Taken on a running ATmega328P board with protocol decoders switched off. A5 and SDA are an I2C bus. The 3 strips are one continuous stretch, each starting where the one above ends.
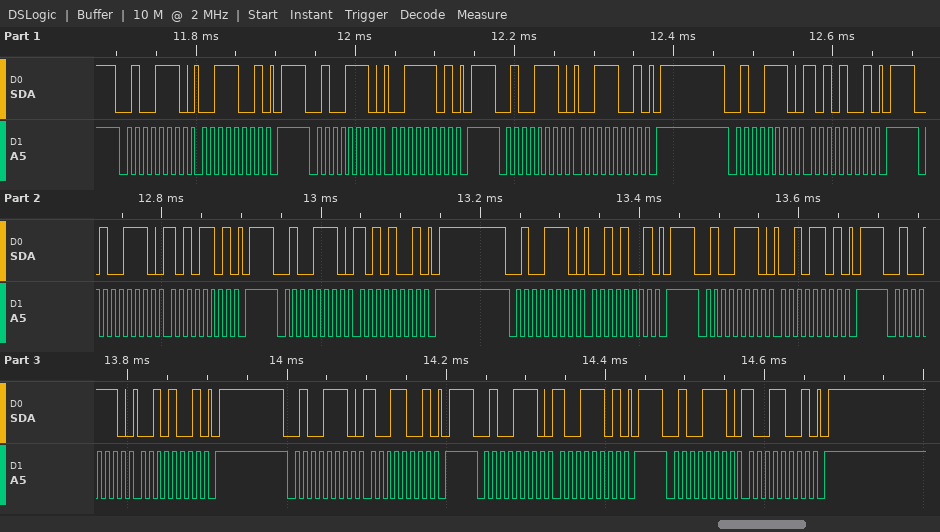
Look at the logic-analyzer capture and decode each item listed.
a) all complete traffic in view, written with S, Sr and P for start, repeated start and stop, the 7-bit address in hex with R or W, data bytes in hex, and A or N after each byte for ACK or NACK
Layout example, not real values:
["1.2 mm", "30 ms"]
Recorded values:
["S 27W A 39 A P S 27W A 3D A P S 27W A 39 A P S 27W A A9 A P S 27W A AD A P S 27W A A9 A P S 27W A 29 A P S 27W A 2D A P S 27W A 29 A P S 27W A 99 A P S 27W A 9D A P S 27W A 99 A P"]
